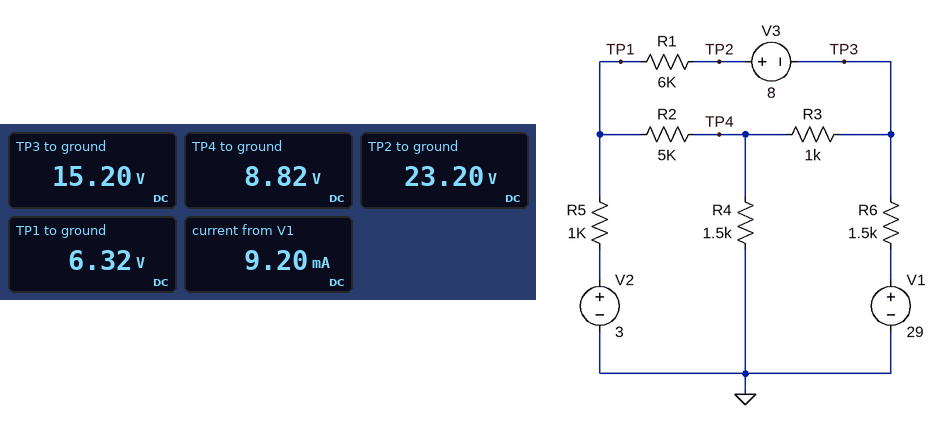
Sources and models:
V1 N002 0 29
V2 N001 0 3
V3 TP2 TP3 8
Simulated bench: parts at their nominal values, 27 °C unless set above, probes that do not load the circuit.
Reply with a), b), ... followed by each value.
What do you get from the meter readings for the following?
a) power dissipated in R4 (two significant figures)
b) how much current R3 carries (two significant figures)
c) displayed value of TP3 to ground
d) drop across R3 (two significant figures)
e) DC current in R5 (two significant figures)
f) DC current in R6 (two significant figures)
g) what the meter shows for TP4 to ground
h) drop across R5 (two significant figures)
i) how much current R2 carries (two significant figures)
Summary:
a) 52 mW
b) 6.4 mA
c) 15.20 V
d) 6.4 V
e) 3.3 mA
f) 9.2 mA
g) 8.82 V
h) 3.3 V
i) 500 µA
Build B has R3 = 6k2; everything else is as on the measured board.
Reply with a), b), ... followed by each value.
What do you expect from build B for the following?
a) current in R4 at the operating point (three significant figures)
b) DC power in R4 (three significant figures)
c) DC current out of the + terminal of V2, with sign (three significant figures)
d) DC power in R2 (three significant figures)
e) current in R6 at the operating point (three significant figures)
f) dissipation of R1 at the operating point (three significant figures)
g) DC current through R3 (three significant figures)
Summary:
a) 2.88 mA
b) 12.5 mW
c) -3.22 mA
d) 721 µW
e) 6.11 mA
f) 77.9 mW
g) 2.50 mA
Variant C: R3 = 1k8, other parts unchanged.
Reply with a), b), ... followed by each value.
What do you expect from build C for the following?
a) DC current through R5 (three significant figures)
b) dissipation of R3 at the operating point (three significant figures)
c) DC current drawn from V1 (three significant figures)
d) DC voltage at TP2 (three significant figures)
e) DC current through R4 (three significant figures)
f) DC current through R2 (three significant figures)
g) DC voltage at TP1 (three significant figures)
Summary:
a) 3.29 mA
b) 47.8 mW
c) 8.22 mA
d) 24.7 V
e) 4.93 mA
f) 222 µA
g) 6.29 V
